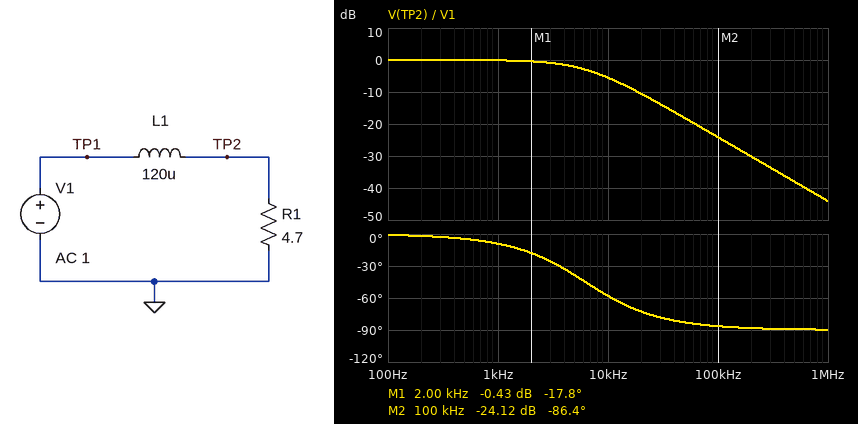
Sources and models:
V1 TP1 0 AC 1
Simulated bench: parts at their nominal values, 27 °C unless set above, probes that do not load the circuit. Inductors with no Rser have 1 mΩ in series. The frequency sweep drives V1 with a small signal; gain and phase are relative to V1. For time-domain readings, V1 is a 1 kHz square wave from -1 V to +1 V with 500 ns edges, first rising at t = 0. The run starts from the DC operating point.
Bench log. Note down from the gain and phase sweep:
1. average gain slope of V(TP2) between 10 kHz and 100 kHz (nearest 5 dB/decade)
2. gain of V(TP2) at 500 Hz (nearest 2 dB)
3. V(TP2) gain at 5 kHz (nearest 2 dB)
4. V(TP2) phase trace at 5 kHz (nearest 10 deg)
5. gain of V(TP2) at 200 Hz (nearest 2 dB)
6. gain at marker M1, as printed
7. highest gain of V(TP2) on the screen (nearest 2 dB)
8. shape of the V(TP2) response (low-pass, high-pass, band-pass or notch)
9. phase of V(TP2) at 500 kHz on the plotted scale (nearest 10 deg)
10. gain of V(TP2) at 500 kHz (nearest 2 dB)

-20 dB/decade
0 dB
-2 dB
-40 deg
0 dB
-0.43 dB
0 dB
low-pass
-90 deg
-38 dB
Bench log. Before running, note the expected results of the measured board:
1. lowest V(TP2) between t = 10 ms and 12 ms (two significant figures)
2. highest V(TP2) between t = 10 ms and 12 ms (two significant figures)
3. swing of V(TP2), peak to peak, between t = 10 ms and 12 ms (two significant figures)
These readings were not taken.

-1.0 V
1.0 V
2.0 V
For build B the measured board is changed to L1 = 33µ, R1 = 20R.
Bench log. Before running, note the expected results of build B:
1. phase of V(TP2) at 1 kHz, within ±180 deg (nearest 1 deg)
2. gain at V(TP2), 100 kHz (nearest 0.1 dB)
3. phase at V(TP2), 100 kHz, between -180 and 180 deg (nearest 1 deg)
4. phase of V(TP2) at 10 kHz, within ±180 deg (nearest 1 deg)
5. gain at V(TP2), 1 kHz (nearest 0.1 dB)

-1 deg
-3.2 dB
-46 deg
-6 deg
0 dB
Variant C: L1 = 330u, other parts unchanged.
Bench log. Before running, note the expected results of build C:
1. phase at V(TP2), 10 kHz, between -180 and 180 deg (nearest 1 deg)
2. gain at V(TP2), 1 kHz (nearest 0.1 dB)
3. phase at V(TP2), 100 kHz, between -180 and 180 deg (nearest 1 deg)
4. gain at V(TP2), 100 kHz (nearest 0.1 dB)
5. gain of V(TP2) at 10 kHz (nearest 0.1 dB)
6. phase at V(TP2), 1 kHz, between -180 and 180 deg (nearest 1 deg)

-77 deg
-0.8 dB
-89 deg
-32.9 dB
-13.1 dB
-24 deg
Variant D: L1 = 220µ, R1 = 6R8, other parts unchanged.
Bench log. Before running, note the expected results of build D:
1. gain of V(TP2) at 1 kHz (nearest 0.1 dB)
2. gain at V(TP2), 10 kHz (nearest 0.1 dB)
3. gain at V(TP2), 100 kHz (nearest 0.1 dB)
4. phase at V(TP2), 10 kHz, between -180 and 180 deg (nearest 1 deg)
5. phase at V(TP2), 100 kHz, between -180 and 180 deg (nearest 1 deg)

-0.2 dB
-7.1 dB
-26.2 dB
-64 deg
-87 deg
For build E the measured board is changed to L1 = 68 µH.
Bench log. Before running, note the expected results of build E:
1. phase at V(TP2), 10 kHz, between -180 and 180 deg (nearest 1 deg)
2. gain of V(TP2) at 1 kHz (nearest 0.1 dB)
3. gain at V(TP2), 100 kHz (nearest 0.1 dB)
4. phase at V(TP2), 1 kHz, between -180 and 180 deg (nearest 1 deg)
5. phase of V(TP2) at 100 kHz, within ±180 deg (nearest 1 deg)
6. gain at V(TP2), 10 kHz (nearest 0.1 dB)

-42 deg
0 dB
-19.2 dB
-5 deg
-84 deg
-2.6 dB
